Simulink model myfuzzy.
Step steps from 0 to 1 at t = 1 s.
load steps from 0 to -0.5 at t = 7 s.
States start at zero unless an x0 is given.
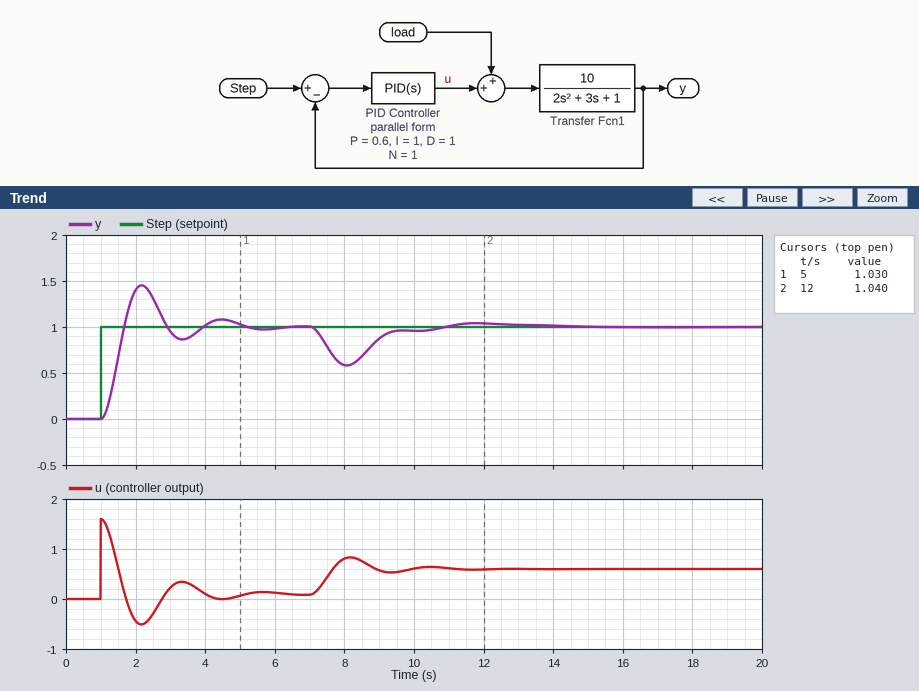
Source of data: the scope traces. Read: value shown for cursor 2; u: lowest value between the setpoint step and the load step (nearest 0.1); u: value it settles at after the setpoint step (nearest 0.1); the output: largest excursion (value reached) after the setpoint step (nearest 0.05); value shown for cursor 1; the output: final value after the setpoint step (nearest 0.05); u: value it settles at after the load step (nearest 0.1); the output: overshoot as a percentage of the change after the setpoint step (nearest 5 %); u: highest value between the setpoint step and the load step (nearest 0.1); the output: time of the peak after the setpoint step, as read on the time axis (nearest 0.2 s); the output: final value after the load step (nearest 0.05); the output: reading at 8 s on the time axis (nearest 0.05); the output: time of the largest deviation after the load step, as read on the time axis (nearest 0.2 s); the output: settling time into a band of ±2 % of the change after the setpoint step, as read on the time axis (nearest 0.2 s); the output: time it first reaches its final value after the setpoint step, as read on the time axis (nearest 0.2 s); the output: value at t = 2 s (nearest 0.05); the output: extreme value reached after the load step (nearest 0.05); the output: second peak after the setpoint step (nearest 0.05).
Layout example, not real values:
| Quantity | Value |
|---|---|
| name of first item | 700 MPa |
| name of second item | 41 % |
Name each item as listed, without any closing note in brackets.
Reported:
| Quantity | Value |
|---|---|
| value shown for cursor 2 | 1.040 |
| u: lowest value between the setpoint step and the load step | -0.5 |
| u: value it settles at after the setpoint step | 0.1 |
| the output: largest excursion (value reached) after the setpoint step | 1.45 |
| value shown for cursor 1 | 1.030 |
| the output: final value after the setpoint step | 1.00 |
| u: value it settles at after the load step | 0.6 |
| the output: overshoot as a percentage of the change after the setpoint step | 45 % |
| u: highest value between the setpoint step and the load step | 1.6 |
| the output: time of the peak after the setpoint step, as read on the time axis | 2.2 s |
| the output: final value after the load step | 1.00 |
| the output: reading at 8 s on the time axis | 0.60 |
| the output: time of the largest deviation after the load step, as read on the time axis | 8.0 s |
| the output: settling time into a band of ±2 % of the change after the setpoint step, as read on the time axis | 6.0 s |
| the output: time it first reaches its final value after the setpoint step, as read on the time axis | 1.6 s |
| the output: value at t = 2 s | 1.40 |
| the output: extreme value reached after the load step | 0.60 |
| the output: second peak after the setpoint step | 1.10 |
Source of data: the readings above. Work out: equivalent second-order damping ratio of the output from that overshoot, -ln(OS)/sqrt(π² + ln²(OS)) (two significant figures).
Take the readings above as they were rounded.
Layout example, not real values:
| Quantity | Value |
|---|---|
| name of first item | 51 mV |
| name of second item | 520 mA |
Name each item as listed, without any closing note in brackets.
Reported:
| Quantity | Value |
|---|---|
| equivalent second-order damping ratio of the output from that overshoot, -ln(OS)/sqrt(π² + ln²(OS)) | 0.25 |
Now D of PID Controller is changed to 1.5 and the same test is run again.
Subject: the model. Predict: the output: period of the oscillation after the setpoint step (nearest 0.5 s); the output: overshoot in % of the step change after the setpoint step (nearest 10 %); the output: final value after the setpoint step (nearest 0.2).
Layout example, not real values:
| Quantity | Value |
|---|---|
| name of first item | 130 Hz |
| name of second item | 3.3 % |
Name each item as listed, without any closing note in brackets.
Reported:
| Quantity | Value |
|---|---|
| the output: period of the oscillation after the setpoint step | 2.0 s |
| the output: overshoot in % of the step change after the setpoint step | 40 % |
| the output: final value after the setpoint step | 1.0 |
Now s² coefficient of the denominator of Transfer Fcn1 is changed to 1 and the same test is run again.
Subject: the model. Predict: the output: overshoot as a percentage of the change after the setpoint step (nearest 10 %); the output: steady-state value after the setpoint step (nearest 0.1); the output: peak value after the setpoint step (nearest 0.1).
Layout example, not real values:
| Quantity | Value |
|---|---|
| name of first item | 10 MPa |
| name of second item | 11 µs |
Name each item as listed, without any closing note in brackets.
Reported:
| Quantity | Value |
|---|---|
| the output: overshoot as a percentage of the change after the setpoint step | 30 % |
| the output: steady-state value after the setpoint step | 1.0 |
| the output: peak value after the setpoint step | 1.3 |
